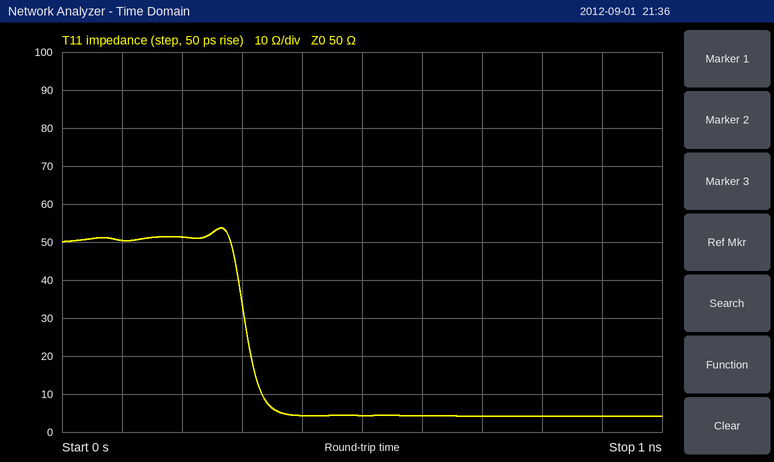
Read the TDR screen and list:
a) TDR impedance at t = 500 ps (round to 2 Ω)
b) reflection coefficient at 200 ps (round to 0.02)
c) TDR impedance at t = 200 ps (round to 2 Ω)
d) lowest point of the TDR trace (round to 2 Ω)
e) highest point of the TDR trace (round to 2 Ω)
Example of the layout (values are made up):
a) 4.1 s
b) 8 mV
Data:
a) 4 Ω
b) +0.02
c) 52 Ω
d) 4 Ω
e) 54 Ω
